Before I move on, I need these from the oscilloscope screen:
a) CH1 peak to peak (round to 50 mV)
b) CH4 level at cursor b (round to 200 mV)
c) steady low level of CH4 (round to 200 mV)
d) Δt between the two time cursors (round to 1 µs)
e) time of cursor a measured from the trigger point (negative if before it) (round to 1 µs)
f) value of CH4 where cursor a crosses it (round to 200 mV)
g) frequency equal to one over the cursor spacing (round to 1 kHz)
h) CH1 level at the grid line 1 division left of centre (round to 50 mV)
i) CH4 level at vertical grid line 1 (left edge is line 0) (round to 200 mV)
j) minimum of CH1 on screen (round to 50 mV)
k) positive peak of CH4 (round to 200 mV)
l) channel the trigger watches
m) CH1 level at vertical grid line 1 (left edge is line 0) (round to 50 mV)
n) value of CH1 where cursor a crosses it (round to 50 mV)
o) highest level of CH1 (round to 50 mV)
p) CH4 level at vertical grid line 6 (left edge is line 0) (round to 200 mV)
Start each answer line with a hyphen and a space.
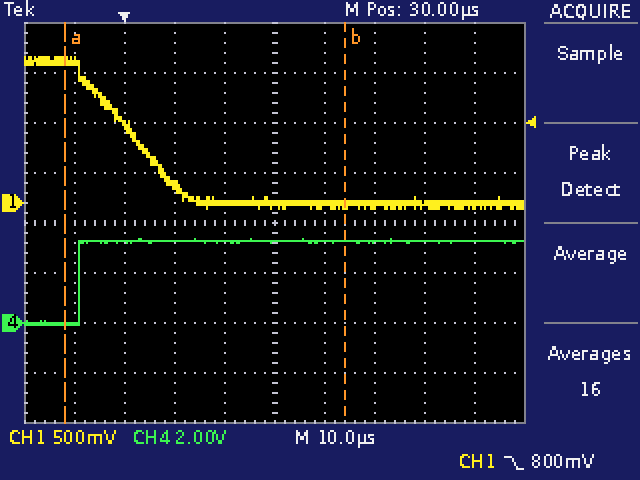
- 1.50 V
- 3.2 V
- 0.0 V
- 56 µs
- -12 µs
- 0.0 V
- 18 kHz
- 0 mV
- 0.0 V
- -50 mV
- 3.4 V
- CH1
- 1.40 V
- 1.40 V
- 1.45 V
- 3.2 V
